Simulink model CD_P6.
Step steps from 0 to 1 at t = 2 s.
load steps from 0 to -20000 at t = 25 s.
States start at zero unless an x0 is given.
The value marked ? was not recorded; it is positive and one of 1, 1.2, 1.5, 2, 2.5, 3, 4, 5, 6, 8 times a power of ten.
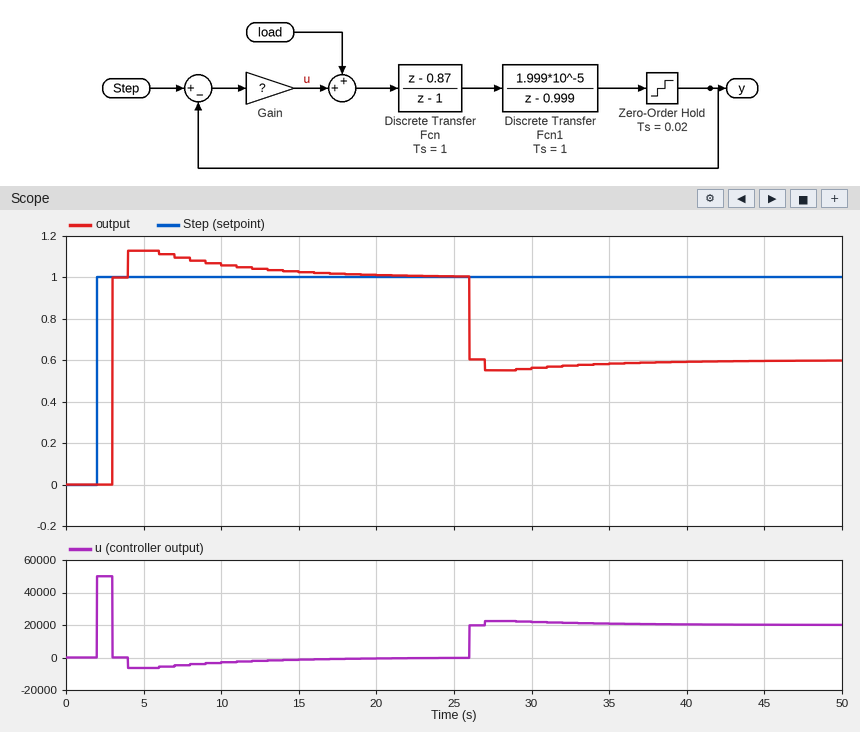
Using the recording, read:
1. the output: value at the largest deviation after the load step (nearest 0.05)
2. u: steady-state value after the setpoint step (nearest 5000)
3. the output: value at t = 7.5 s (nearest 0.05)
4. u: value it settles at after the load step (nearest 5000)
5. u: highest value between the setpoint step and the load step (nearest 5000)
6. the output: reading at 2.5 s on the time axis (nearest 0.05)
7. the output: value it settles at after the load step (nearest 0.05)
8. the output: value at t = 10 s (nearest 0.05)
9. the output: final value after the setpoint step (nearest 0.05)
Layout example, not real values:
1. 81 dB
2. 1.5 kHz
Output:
1. 0.55
2. 0
3. 1.10
4. 20000
5. 50000
6. 0.00
7. 0.60
8. 1.05
9. 1.00
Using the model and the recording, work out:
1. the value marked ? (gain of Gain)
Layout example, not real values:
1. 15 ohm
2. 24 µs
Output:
1. 50000
